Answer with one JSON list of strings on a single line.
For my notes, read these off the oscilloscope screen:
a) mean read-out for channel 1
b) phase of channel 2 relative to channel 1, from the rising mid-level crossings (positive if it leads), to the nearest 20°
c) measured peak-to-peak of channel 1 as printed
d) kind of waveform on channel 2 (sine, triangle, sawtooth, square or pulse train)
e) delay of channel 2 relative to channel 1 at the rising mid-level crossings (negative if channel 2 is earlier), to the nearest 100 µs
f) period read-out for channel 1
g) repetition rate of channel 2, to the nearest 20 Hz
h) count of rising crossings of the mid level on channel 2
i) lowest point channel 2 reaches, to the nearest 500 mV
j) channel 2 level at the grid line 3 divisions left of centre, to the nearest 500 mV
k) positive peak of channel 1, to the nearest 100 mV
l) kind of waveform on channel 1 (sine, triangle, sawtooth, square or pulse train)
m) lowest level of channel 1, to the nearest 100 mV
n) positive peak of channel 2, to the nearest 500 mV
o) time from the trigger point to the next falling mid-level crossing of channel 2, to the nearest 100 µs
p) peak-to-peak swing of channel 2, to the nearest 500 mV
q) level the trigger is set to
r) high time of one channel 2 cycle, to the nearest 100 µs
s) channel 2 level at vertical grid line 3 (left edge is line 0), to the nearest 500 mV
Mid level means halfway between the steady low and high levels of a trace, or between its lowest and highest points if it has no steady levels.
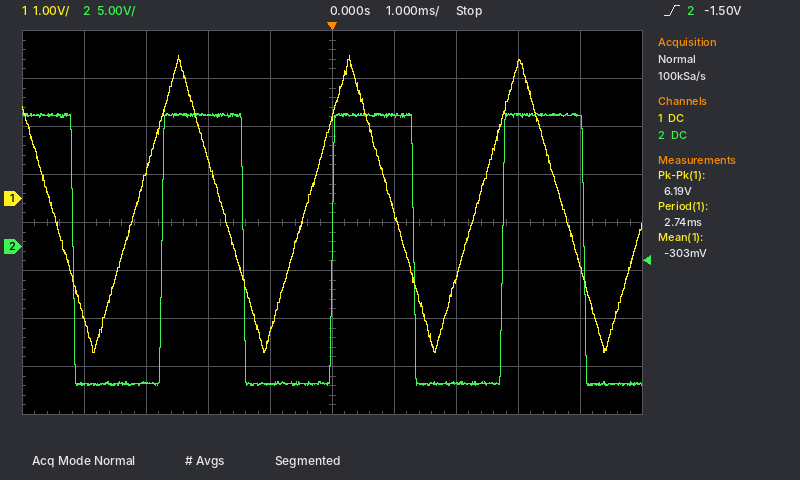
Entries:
["-303 mV", "-60°", "6.19 V", "square", "+400 µs", "2.74 ms", "360 Hz", "3", "-14.5 V", "-14.0 V", "3.0 V", "triangle", "-3.2 V", "14.0 V", "1.3 ms", "28.5 V", "-1.50 V", "1.3 ms", "13.5 V"]
